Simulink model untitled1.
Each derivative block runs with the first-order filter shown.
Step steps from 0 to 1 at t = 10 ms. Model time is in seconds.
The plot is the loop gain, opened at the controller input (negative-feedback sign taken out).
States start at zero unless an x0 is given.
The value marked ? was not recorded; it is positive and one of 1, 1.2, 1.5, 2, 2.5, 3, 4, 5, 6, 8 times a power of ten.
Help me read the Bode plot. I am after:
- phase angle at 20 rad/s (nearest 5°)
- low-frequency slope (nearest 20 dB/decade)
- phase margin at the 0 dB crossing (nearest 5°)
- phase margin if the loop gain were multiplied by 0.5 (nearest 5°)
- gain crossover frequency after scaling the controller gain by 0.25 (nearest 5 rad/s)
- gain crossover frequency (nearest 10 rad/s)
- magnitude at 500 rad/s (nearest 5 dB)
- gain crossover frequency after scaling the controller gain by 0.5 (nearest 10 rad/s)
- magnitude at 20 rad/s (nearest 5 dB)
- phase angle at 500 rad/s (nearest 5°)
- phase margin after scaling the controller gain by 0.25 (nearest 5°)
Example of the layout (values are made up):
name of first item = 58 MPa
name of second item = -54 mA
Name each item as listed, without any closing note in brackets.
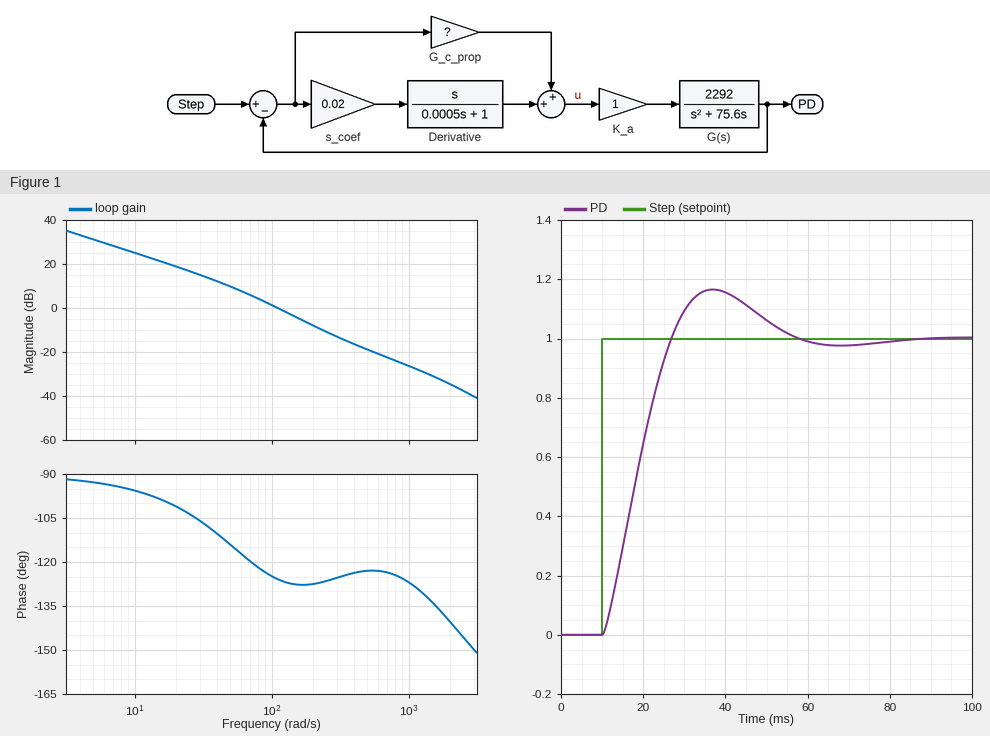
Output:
phase angle at 20 rad/s = -100°
low-frequency slope = -20 dB/decade
phase margin at the 0 dB crossing = 55°
phase margin if the loop gain were multiplied by 0.5 = 60°
gain crossover frequency after scaling the controller gain by 0.25 = 40 rad/s
gain crossover frequency = 110 rad/s
magnitude at 500 rad/s = -20 dB
gain crossover frequency after scaling the controller gain by 0.5 = 70 rad/s
magnitude at 20 rad/s = 20 dB
phase angle at 500 rad/s = -125°
phase margin after scaling the controller gain by 0.25 = 70°
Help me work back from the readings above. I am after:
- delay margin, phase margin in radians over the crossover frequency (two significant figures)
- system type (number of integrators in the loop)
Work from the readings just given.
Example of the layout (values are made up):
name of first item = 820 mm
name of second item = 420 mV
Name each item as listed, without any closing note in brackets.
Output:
delay margin, phase margin in radians over the crossover frequency = 0.0087 s
system type = 1
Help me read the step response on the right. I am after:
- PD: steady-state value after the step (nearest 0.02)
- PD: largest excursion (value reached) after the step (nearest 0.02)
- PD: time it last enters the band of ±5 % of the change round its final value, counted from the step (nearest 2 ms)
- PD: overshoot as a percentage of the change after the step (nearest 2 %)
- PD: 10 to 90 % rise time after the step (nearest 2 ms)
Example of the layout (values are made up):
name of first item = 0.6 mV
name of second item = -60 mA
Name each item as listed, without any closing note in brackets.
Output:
PD: steady-state value after the step = 1.00
PD: largest excursion (value reached) after the step = 1.16
PD: time it last enters the band of ±5 % of the change round its final value, counted from the step = 42 ms
PD: overshoot as a percentage of the change after the step = 16 %
PD: 10 to 90 % rise time after the step = 12 ms
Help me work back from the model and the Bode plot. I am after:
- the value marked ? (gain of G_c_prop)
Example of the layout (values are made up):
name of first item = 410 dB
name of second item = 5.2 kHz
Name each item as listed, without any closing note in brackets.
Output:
the value marked ? = 6
